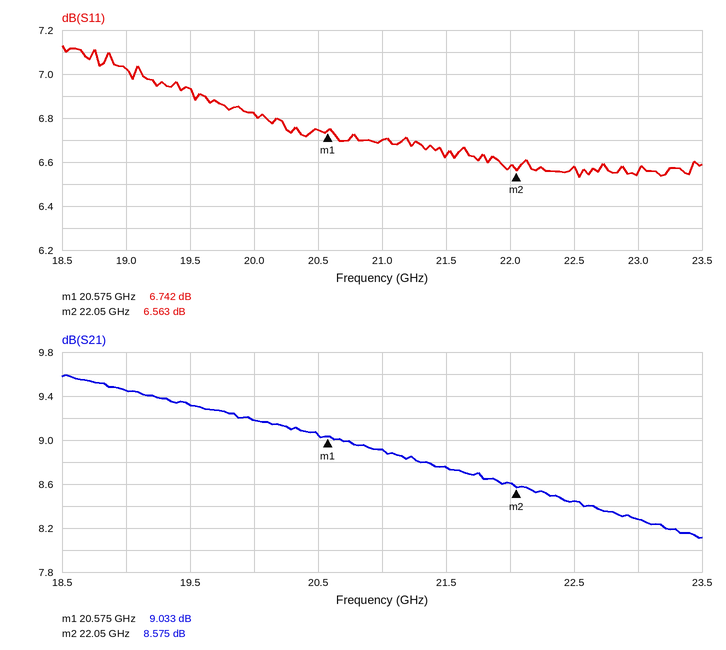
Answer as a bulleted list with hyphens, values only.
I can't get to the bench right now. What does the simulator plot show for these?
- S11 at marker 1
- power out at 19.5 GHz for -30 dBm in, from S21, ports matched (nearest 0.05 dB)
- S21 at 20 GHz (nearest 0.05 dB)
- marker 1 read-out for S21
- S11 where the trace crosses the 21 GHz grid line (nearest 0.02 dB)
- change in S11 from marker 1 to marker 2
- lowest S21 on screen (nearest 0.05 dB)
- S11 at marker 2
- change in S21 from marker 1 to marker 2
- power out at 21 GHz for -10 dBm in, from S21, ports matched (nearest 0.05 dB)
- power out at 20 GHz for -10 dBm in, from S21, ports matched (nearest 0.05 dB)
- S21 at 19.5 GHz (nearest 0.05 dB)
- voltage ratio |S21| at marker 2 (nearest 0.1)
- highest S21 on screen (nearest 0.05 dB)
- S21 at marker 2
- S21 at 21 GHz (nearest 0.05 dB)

- 6.742 dB
- -20.70 dBm
- 9.20 dB
- 9.033 dB
- 6.70 dB
- -0.179 dB
- 8.10 dB
- 6.563 dB
- -0.458 dB
- -1.10 dBm
- -0.80 dBm
- 9.30 dB
- 2.7
- 9.60 dB
- 8.575 dB
- 8.90 dB
